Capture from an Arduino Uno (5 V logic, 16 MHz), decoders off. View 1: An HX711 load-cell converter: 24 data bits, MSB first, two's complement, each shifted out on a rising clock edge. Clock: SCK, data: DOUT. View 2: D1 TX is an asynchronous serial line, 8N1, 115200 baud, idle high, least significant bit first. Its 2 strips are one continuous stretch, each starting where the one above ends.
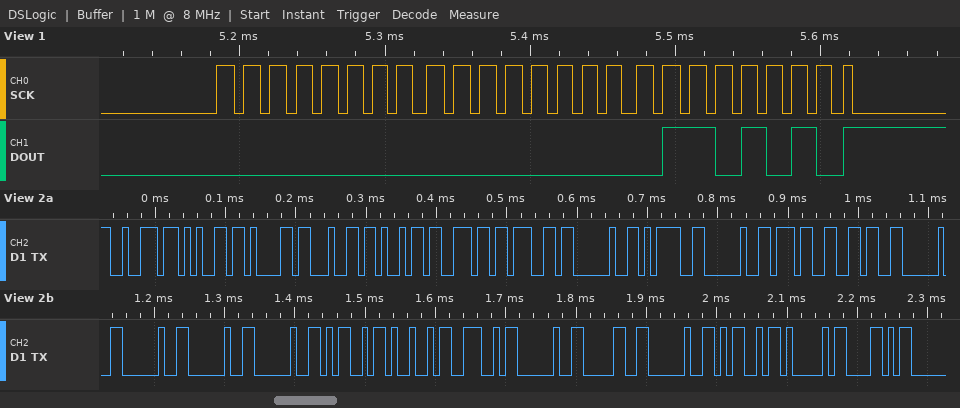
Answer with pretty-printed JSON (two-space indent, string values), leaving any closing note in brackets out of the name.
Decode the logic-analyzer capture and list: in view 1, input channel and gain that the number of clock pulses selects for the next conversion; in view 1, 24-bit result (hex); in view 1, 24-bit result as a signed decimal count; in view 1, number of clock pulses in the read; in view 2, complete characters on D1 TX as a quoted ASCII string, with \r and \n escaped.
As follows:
{
  "in view 1, input channel and gain that the number of clock pulses selects for the next conversion": "channel A, gain 128",
  "in view 1, 24-bit result": "0x00006A",
  "in view 1, 24-bit result as a signed decimal count": "106",
  "in view 1, number of clock pulses in the read": "25",
  "in view 2, complete characters on D1 TX as a quoted ASCII string, with \\r and \\n escaped": "\"reading = 76    MIN 0 MAX\""
}
